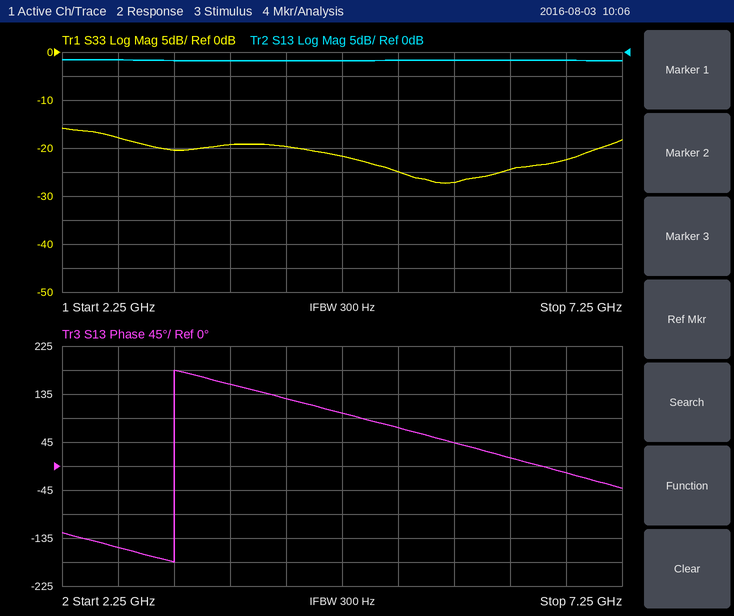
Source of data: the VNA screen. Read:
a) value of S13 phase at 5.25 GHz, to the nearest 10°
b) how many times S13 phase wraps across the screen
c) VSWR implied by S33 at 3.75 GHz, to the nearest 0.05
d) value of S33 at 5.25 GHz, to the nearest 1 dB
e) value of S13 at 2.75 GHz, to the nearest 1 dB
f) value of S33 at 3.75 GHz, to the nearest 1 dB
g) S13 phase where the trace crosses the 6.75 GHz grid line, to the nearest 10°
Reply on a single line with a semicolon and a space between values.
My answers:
70°; 1; 1.25; -25 dB; -2 dB; -19 dB; -10°
